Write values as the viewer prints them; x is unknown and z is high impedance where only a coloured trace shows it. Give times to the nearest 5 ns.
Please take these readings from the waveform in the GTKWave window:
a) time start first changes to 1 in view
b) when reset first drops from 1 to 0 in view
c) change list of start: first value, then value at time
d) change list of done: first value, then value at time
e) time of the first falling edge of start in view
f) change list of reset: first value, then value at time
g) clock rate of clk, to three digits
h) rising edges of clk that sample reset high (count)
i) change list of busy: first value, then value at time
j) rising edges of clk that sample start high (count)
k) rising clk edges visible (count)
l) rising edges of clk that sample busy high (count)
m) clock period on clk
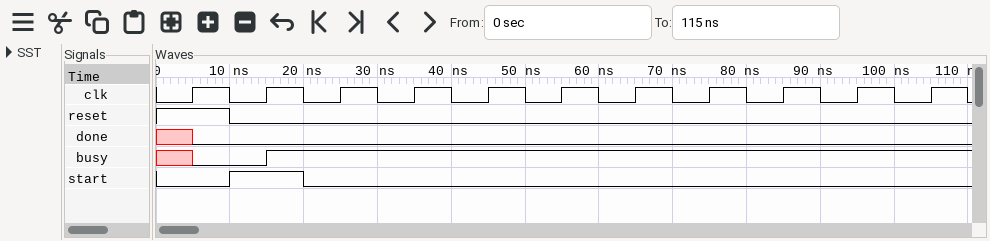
10 ns
10 ns
0, 1 at 10 ns, 0 at 20 ns
x, 0 at 5 ns
20 ns
1, 0 at 10 ns
100 MHz
1
x, 0 at 5 ns, 1 at 15 ns
1
11
9
10 ns
